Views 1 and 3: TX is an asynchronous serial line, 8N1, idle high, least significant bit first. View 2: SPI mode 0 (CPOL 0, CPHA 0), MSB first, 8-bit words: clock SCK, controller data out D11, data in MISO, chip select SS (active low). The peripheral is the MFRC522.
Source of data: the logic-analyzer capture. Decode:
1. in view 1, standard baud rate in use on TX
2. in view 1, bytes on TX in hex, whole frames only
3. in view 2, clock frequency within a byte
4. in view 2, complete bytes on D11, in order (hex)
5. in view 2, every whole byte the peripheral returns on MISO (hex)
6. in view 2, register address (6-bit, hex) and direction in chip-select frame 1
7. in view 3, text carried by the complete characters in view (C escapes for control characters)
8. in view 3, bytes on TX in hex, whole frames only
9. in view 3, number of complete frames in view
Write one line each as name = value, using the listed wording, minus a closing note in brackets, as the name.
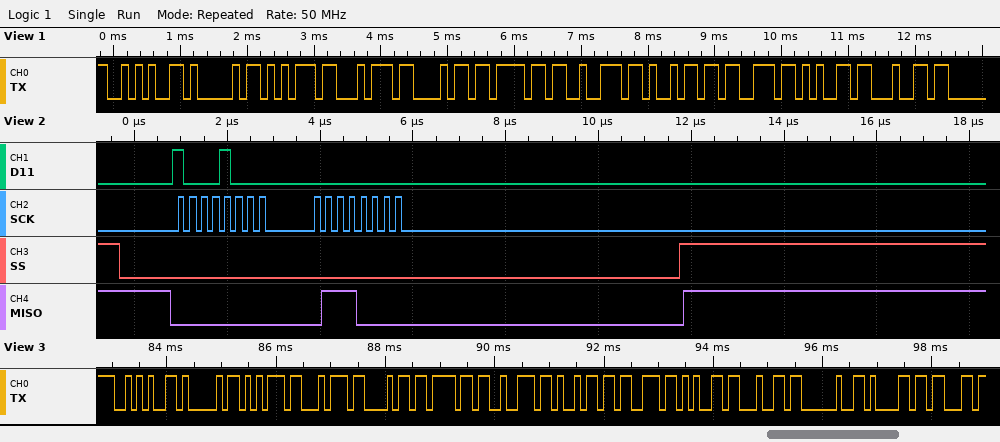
in view 1, standard baud rate in use on TX = 9600 baud
in view 1, bytes on TX in hex, whole frames only = 2A 41 75 74 68 6F 72 69 73 65 64
in view 2, clock frequency within a byte = 4 MHz
in view 2, complete bytes on D11, in order = 88 00
in view 2, every whole byte the peripheral returns on MISO = 00 70
in view 2, register address (6-bit, hex) and direction in chip-select frame 1 = 0x04 read
in view 3, text carried by the complete characters in view = "*Authorised ac"
in view 3, bytes on TX in hex, whole frames only = 2A 41 75 74 68 6F 72 69 73 65 64 20 61 63
in view 3, number of complete frames in view = 14
